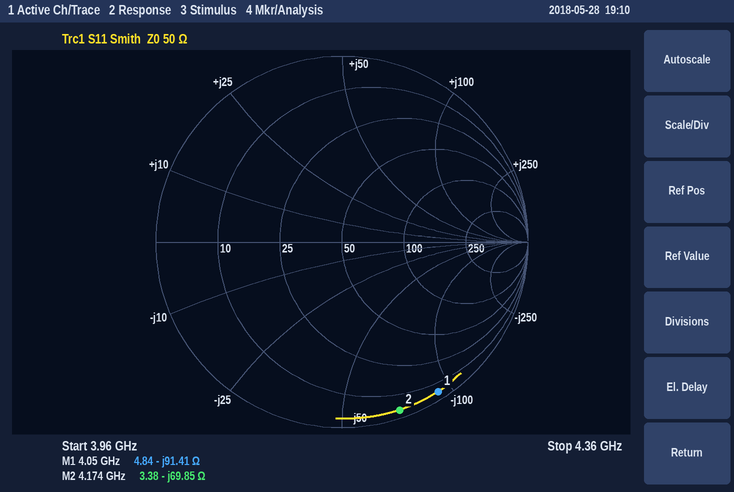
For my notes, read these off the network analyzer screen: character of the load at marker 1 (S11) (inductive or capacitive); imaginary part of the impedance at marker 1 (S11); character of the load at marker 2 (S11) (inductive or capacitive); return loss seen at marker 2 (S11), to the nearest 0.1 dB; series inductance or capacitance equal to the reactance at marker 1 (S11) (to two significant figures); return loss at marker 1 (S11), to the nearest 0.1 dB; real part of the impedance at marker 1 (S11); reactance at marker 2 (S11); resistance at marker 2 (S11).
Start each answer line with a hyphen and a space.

- capacitive
- -91.41 Ω
- capacitive
- 0.4 dB
- 430 fF
- 0.4 dB
- 4.84 Ω
- -69.85 Ω
- 3.38 Ω
